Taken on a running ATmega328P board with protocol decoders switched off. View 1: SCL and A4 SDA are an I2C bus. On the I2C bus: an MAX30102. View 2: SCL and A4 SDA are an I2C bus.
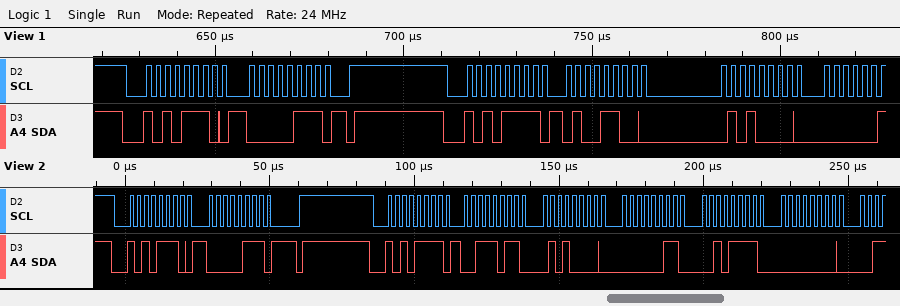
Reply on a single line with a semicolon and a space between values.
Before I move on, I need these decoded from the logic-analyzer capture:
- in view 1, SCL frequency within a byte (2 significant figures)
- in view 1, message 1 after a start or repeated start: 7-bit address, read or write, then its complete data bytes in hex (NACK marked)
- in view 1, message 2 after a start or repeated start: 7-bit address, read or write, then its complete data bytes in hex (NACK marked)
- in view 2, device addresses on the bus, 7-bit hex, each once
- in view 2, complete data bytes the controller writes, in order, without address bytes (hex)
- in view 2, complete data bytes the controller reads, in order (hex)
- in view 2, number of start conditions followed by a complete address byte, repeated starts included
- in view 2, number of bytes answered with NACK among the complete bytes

400 kHz; 0x57 write: 07; 0x57 read: 4C 50; 0x57; 07; 3B 50 03 2F 00; 2; 0
